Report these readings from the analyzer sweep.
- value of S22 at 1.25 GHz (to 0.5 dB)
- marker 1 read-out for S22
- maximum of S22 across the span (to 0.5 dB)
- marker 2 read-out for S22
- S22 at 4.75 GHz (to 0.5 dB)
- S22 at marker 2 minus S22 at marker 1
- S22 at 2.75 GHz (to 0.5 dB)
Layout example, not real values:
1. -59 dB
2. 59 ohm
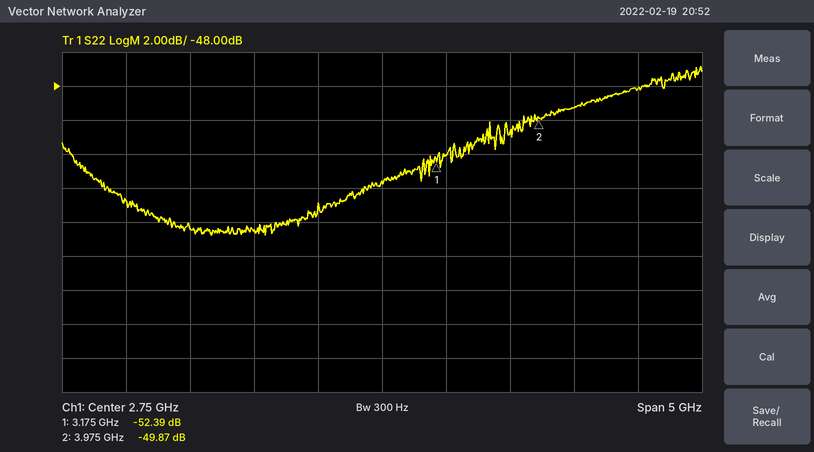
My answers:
1. -56.5 dB
2. -52.39 dB
3. -47.0 dB
4. -49.87 dB
5. -48.0 dB
6. 2.52 dB
7. -53.5 dB
